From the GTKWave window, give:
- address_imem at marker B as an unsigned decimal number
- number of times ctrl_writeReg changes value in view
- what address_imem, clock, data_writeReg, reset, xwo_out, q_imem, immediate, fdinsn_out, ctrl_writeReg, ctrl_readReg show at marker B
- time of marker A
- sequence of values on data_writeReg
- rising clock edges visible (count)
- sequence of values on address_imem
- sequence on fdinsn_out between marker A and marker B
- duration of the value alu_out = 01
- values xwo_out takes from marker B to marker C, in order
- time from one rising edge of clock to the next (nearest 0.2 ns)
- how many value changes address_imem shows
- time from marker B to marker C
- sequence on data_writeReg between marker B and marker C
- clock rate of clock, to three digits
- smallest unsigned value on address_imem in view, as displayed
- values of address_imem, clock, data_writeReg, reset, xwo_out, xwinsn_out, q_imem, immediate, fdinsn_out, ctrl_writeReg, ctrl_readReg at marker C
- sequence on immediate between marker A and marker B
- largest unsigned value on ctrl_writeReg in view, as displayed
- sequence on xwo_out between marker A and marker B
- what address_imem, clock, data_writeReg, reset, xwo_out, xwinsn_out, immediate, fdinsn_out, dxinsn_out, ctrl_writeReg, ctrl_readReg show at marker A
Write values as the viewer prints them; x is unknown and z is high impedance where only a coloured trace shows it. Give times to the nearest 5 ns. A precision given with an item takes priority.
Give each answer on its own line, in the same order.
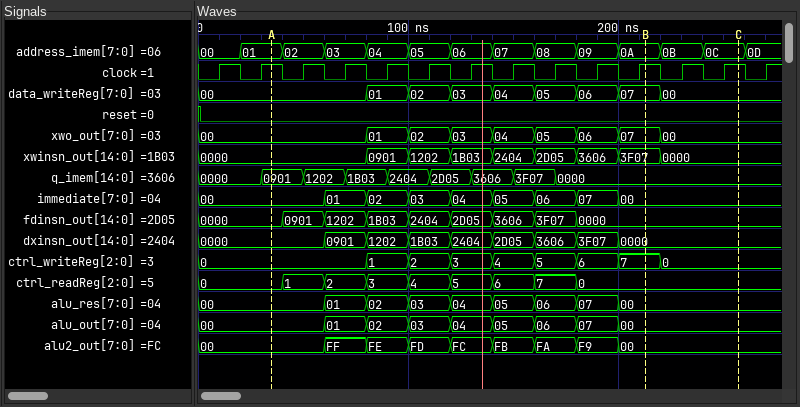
10
8
address_imem=0A, clock=1, data_writeReg=07, reset=0, xwo_out=07, q_imem=0000, immediate=00, fdinsn_out=0000, ctrl_writeReg=7, ctrl_readReg=0
35 ns
00, 01, 02, 03, 04, 05, 06, 07, 00
14
00, 01, 02, 03, 04, 05, 06, 07, 08, 09, 0A, 0B, 0C, 0D
0000, 0901, 1202, 1B03, 2404, 2D05, 3606, 3F07, 0000
20 ns
07, 00
20 ns
13
45 ns
07, 00
50.0 MHz
00
address_imem=0C, clock=1, data_writeReg=00, reset=0, xwo_out=00, xwinsn_out=0000, q_imem=0000, immediate=00, fdinsn_out=0000, ctrl_writeReg=0, ctrl_readReg=0
00, 01, 02, 03, 04, 05, 06, 07, 00
7
00, 01, 02, 03, 04, 05, 06, 07
address_imem=01, clock=1, data_writeReg=00, reset=0, xwo_out=00, xwinsn_out=0000, immediate=00, fdinsn_out=0000, dxinsn_out=0000, ctrl_writeReg=0, ctrl_readReg=0
